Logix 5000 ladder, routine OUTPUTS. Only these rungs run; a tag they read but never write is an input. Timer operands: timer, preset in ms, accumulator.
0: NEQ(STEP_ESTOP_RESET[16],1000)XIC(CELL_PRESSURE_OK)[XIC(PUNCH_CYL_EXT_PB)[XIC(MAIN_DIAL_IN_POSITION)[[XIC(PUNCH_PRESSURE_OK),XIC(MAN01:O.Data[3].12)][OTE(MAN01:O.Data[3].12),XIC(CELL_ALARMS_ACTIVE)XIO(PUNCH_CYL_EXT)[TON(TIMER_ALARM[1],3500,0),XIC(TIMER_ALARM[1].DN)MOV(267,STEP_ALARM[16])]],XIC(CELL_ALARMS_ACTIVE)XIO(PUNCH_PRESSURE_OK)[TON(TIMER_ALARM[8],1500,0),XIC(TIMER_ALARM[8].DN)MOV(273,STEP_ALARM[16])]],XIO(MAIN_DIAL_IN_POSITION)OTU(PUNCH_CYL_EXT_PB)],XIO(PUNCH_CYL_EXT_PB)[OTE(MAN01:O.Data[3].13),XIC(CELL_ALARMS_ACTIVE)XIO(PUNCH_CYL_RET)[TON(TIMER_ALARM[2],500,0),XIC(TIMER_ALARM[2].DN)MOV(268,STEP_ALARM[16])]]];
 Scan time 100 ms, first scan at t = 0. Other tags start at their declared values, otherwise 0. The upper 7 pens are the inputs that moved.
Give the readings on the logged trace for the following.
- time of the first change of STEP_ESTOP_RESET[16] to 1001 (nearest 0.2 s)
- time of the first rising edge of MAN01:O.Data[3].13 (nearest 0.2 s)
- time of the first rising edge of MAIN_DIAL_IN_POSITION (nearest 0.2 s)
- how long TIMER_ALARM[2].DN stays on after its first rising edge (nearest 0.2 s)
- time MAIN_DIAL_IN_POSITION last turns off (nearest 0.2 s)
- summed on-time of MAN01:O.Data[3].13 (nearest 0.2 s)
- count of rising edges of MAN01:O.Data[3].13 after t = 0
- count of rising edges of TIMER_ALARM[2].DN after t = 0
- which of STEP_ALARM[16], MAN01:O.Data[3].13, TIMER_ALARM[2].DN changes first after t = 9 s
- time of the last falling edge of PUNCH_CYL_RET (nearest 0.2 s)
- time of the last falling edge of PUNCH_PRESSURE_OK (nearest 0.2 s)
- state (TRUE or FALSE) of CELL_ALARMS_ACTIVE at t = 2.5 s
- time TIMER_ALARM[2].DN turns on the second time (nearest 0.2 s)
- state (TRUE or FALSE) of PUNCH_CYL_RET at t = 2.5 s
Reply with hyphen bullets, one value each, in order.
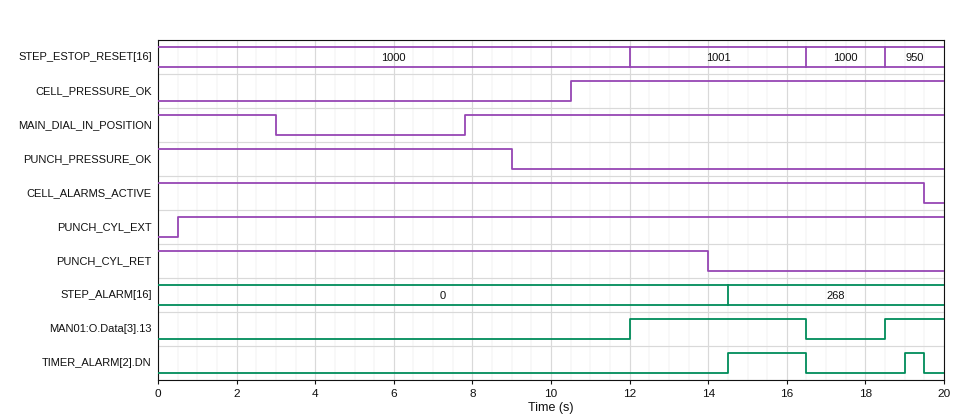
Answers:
- 12.0 s
- 12.0 s
- 7.8 s
- 2.0 s
- 3.0 s
- 6.0 s
- 2
- 2
- MAN01:O.Data[3].13
- 14.0 s
- 9.0 s
- TRUE
- 19.0 s
- TRUE
